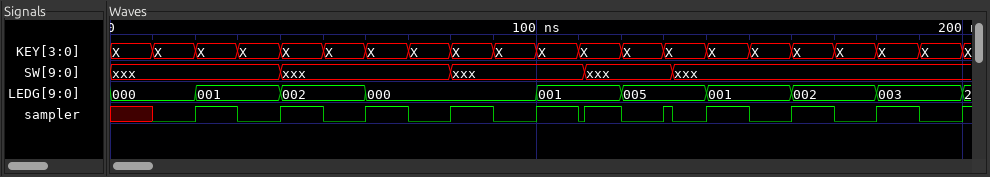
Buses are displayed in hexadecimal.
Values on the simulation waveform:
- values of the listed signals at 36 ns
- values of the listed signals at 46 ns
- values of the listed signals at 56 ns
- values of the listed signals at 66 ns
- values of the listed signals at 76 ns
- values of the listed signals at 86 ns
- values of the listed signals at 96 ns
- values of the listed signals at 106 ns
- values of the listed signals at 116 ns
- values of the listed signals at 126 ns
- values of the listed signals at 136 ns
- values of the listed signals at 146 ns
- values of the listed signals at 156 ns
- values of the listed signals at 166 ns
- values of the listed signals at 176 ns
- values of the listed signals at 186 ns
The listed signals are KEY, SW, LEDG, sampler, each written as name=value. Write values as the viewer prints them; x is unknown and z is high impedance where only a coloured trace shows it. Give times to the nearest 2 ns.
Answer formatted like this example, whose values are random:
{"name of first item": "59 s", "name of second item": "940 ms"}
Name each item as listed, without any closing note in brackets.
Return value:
{"values of the listed signals at 36 ns": "KEY=X, SW=xxx, LEDG=001, sampler=0", "values of the listed signals at 46 ns": "KEY=X, SW=xxx, LEDG=002, sampler=1", "values of the listed signals at 56 ns": "KEY=X, SW=xxx, LEDG=002, sampler=0", "values of the listed signals at 66 ns": "KEY=X, SW=xxx, LEDG=000, sampler=1", "values of the listed signals at 76 ns": "KEY=X, SW=xxx, LEDG=000, sampler=0", "values of the listed signals at 86 ns": "KEY=X, SW=xxx, LEDG=000, sampler=1", "values of the listed signals at 96 ns": "KEY=X, SW=xxx, LEDG=000, sampler=0", "values of the listed signals at 106 ns": "KEY=X, SW=xxx, LEDG=001, sampler=1", "values of the listed signals at 116 ns": "KEY=X, SW=xxx, LEDG=001, sampler=1", "values of the listed signals at 126 ns": "KEY=X, SW=xxx, LEDG=005, sampler=0", "values of the listed signals at 136 ns": "KEY=X, SW=xxx, LEDG=005, sampler=0", "values of the listed signals at 146 ns": "KEY=X, SW=xxx, LEDG=001, sampler=1", "values of the listed signals at 156 ns": "KEY=X, SW=xxx, LEDG=001, sampler=0", "values of the listed signals at 166 ns": "KEY=X, SW=xxx, LEDG=002, sampler=1", "values of the listed signals at 176 ns": "KEY=X, SW=xxx, LEDG=002, sampler=0", "values of the listed signals at 186 ns": "KEY=X, SW=xxx, LEDG=003, sampler=1"}
